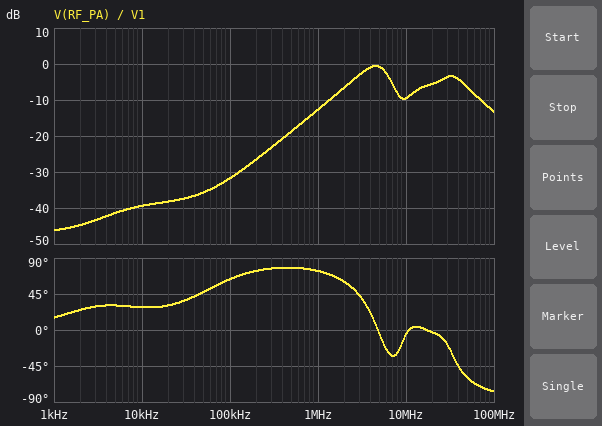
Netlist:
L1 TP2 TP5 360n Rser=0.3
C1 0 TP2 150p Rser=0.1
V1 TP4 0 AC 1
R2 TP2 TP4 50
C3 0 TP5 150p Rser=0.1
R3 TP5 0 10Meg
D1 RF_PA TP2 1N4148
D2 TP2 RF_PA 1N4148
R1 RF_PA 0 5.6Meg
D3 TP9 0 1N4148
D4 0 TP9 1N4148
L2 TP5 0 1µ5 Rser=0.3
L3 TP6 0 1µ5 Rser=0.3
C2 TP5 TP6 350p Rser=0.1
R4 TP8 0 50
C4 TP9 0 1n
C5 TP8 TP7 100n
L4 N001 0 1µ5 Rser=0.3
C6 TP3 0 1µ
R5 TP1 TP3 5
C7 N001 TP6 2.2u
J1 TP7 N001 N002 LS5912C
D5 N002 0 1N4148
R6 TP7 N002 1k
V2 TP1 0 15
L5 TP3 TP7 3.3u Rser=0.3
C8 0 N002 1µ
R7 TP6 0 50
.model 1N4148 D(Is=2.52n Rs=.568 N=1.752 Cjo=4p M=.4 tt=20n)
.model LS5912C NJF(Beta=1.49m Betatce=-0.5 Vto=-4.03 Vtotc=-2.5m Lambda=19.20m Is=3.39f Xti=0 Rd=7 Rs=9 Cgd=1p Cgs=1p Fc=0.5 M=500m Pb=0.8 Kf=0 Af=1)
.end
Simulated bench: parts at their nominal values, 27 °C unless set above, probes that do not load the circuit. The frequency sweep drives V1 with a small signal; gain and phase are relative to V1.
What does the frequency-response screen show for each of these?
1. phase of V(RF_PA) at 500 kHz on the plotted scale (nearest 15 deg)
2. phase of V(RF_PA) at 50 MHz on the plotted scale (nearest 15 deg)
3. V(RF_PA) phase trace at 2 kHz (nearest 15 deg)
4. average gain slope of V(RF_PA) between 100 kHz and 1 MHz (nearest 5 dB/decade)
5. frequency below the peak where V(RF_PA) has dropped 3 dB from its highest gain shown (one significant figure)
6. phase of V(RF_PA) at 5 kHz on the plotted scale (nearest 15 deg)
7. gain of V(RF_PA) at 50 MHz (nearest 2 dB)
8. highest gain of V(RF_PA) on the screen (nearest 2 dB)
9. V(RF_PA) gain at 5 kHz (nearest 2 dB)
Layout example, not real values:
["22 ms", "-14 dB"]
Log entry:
["75 deg", "-60 deg", "30 deg", "20 dB/decade", "3 MHz", "30 deg", "-6 dB", "0 dB", "-42 dB"]
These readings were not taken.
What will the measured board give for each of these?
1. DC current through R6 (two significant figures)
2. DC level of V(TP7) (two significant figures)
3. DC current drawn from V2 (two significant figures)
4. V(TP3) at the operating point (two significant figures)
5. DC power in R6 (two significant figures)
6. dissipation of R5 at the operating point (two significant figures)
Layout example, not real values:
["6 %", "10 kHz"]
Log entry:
["14 mA", "15 V", "32 mA", "15 V", "200 mW", "5.2 mW"]
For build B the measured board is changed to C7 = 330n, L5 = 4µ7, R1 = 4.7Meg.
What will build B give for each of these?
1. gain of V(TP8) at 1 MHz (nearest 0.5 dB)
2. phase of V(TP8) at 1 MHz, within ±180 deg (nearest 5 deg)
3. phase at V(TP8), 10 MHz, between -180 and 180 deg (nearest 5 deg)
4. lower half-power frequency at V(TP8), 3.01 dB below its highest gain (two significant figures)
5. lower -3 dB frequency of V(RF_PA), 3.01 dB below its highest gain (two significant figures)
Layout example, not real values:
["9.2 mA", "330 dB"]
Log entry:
["-65.5 dB", "125 deg", "-135 deg", "6.2 MHz", "2.8 MHz"]
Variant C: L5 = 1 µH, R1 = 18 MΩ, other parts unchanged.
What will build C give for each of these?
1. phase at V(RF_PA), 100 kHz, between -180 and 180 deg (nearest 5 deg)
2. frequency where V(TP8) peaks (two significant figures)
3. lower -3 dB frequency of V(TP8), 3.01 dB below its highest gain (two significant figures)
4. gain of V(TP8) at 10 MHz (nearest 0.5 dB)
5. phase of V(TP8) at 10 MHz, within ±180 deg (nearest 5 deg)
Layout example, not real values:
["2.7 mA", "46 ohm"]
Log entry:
["60 deg", "22 MHz", "8.4 MHz", "-14.5 dB", "-105 deg"]
